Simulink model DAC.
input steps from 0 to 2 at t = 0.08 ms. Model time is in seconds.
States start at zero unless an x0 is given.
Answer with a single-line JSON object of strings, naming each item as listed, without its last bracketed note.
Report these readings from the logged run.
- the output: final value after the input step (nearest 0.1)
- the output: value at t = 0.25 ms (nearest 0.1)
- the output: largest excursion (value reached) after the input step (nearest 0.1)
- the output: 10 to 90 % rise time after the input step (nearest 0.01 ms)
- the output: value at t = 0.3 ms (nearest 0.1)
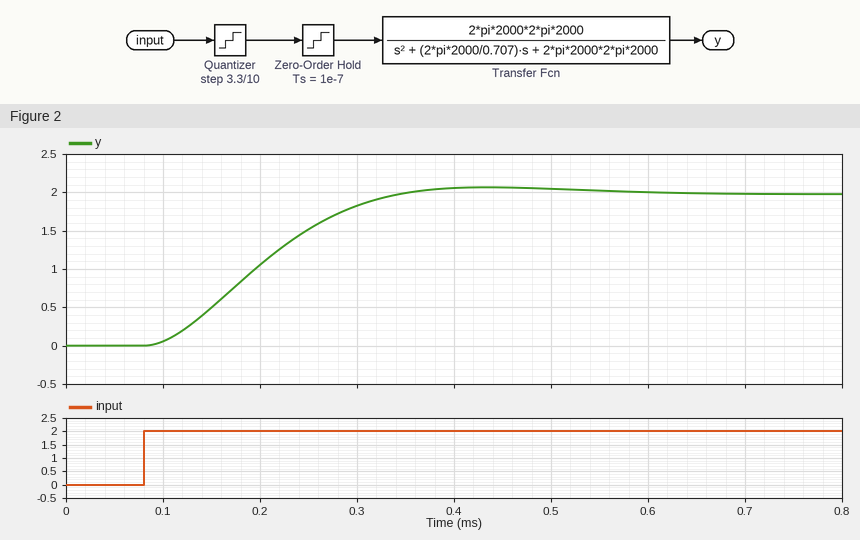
{"the output: final value after the input step": "2.0", "the output: value at t = 0.25 ms": "1.5", "the output: largest excursion (value reached) after the input step": "2.1", "the output: 10 to 90 % rise time after the input step": "0.17 ms", "the output: value at t = 0.3 ms": "1.8"}
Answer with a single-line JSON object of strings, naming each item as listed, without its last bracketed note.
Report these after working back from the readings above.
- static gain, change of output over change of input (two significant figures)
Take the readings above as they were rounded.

{"static gain, change of output over change of input": "1.0"}
